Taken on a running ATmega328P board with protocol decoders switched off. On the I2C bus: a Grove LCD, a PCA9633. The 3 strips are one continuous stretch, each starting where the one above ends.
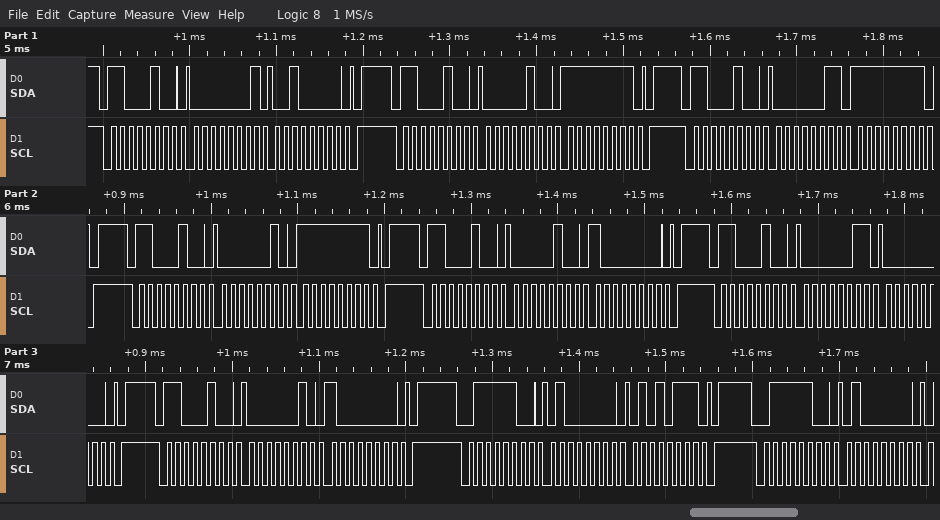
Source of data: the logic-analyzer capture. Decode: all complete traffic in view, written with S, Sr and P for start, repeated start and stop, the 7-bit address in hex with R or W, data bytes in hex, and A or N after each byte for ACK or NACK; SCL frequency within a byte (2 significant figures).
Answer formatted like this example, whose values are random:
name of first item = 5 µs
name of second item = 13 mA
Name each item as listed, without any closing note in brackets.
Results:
all complete traffic in view, written with S, Sr and P for start, repeated start and stop, the 7-bit address in hex with R or W, data bytes in hex, and A or N after each byte for ACK or NACK = S 62W A 01 A 20 A P S 62W A 04 A FF A P S 62W A 03 A FF A P S 62W A 02 A FF A P S 62W A 04 A 80 A P S 62W A 03 A 00 A P S 62W A 02 A 80 A P S 3EW A 40 A 57 A P S 3EW A 40 A
SCL frequency within a byte = 100 kHz
